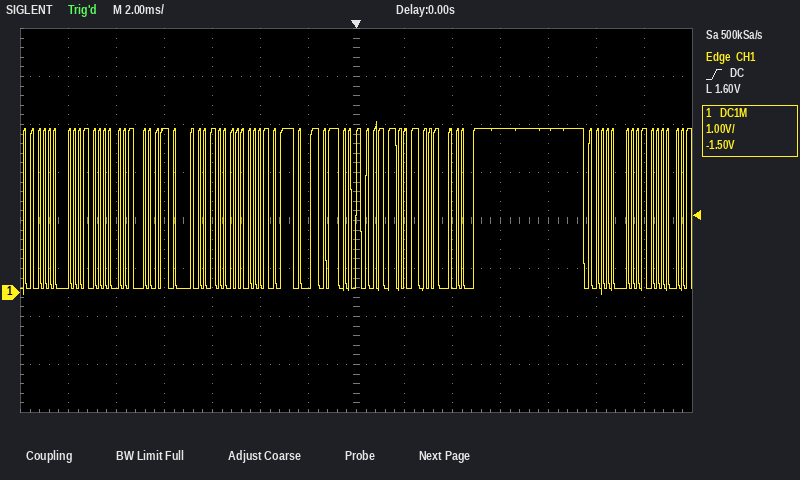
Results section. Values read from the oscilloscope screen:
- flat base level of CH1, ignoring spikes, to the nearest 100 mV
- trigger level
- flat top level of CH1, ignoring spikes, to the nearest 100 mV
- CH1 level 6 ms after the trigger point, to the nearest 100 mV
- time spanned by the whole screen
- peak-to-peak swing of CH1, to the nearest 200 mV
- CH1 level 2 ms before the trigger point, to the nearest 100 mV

100 mV
1.60 V
3.4 V
3.4 V
28 ms
3.6 V
100 mV
